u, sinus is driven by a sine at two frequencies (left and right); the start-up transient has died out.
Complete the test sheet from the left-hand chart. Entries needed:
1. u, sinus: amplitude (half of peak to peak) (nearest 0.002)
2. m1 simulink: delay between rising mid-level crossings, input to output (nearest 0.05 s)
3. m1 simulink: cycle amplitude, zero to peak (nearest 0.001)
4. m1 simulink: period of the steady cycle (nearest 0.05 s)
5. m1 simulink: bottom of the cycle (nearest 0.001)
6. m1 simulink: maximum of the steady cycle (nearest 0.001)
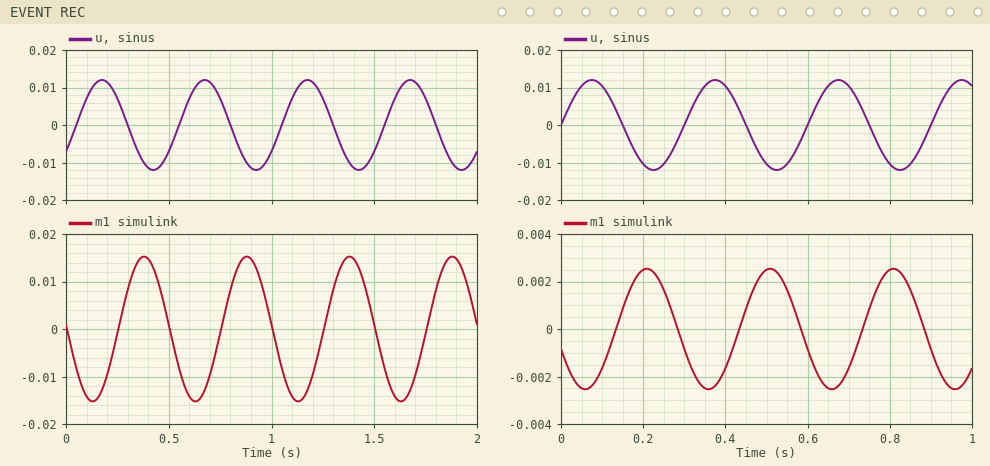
0.012
0.20 s
0.015
0.50 s
-0.015
0.015
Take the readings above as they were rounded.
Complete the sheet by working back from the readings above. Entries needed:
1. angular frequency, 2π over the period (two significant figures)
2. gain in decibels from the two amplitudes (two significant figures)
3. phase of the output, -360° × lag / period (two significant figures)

13 rad/s
1.9 dB
-140°
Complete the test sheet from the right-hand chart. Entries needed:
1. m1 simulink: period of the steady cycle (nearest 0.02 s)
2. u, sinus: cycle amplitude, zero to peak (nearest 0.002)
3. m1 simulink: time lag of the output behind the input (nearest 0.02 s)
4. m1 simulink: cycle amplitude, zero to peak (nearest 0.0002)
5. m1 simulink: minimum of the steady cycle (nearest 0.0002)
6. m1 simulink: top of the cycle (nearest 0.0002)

0.30 s
0.012
0.14 s
0.0026
-0.0026
0.0026
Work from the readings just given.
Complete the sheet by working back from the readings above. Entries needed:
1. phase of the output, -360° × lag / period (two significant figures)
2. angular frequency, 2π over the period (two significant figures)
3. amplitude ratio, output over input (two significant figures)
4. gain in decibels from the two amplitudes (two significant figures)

-170°
21 rad/s
0.22
-13 dB
